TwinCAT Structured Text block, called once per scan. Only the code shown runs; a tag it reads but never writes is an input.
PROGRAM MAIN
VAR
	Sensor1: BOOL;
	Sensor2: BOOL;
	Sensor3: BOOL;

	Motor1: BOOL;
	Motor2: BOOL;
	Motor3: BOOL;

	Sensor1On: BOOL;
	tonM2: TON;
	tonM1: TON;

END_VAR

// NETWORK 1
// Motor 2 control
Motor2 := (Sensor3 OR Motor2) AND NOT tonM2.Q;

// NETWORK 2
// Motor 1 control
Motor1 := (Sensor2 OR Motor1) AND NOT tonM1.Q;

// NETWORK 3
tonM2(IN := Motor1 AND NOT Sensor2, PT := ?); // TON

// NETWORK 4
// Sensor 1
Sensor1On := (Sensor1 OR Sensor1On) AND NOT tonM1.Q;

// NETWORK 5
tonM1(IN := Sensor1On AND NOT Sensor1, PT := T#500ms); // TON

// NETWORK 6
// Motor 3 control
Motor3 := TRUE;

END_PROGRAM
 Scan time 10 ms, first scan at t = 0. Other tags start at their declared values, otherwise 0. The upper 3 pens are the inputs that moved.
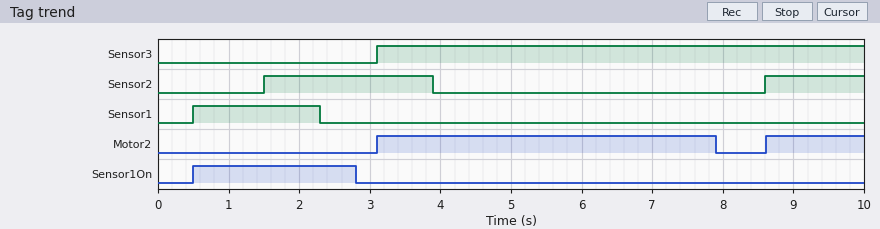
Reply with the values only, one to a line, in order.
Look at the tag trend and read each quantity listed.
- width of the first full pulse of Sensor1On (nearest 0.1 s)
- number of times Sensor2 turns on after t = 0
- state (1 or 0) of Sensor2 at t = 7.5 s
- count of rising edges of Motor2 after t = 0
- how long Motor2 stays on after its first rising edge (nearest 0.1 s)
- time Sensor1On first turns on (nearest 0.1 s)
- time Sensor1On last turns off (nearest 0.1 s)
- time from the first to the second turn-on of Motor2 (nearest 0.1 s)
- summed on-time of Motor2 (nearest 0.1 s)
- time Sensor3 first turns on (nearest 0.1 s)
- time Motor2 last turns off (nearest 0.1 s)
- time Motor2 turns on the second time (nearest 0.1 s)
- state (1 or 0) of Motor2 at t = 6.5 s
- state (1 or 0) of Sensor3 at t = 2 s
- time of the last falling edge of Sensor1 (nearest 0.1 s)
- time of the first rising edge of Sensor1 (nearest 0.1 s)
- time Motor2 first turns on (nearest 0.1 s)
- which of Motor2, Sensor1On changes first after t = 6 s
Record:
2.3 s
2
0
2
4.8 s
0.5 s
2.8 s
5.5 s
6.2 s
3.1 s
7.9 s
8.6 s
1
0
2.3 s
0.5 s
3.1 s
Motor2
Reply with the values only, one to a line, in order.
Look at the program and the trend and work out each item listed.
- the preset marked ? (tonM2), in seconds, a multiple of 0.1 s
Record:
4.0 s
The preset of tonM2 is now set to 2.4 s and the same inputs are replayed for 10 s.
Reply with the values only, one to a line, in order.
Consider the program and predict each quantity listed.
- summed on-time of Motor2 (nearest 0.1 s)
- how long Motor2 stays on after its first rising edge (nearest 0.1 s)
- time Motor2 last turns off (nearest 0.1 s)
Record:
4.6 s
3.2 s
6.3 s
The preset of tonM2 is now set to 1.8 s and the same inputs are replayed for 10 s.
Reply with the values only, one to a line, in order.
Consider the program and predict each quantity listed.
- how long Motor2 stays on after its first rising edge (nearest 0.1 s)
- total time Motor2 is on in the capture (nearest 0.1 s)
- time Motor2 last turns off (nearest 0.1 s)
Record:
2.6 s
4.0 s
5.7 s
